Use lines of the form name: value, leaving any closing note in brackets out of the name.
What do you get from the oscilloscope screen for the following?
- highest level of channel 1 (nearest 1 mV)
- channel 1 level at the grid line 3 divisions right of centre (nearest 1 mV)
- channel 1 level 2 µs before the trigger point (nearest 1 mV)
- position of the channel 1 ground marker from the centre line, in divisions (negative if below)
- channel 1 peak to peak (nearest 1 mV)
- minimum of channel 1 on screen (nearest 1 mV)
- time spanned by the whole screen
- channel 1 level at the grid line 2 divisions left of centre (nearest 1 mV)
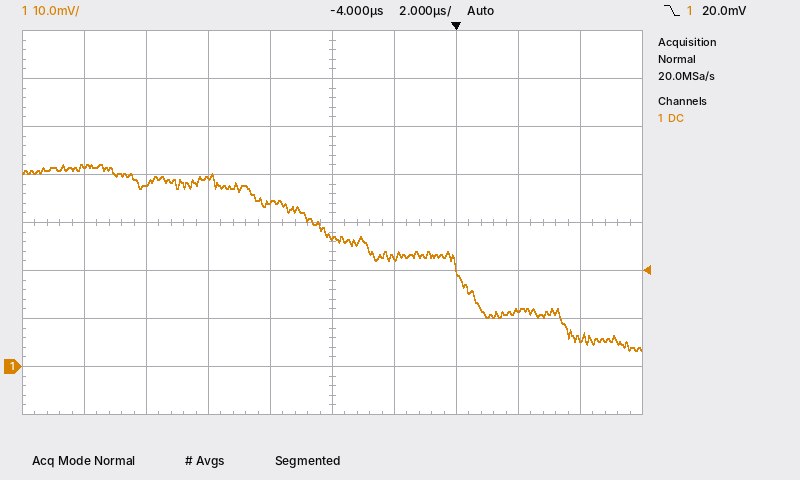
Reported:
highest level of channel 1: 42 mV
channel 1 level at the grid line 3 divisions right of centre: 12 mV
channel 1 level 2 µs before the trigger point: 23 mV
position of the channel 1 ground marker from the centre line, in divisions: -3.0 div
channel 1 peak to peak: 39 mV
minimum of channel 1 on screen: 3 mV
time spanned by the whole screen: 20 µs
channel 1 level at the grid line 2 divisions left of centre: 39 mV
